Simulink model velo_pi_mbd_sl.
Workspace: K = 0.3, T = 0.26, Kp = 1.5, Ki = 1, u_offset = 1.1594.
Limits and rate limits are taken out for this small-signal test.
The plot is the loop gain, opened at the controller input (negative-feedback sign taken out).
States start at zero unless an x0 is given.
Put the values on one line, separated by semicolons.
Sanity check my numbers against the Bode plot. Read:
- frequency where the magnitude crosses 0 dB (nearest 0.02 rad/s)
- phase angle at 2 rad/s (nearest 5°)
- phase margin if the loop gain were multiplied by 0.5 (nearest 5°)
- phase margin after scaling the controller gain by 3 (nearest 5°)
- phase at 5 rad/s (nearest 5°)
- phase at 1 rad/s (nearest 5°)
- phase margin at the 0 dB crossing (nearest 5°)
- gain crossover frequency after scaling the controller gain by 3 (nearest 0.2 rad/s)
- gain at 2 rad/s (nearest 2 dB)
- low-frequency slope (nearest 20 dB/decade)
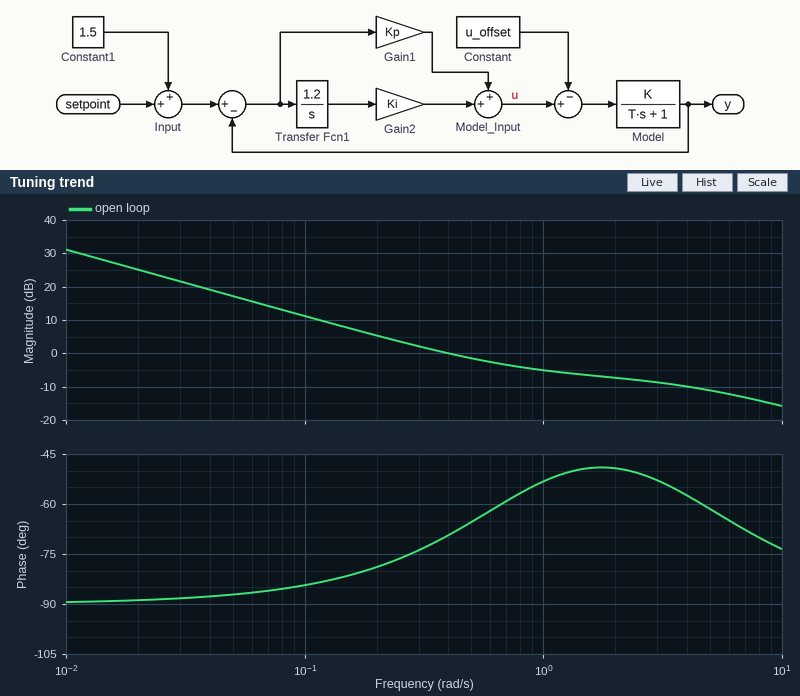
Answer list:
0.40 rad/s; -50°; 100°; 125°; -60°; -55°; 110°; 3.6 rad/s; -8 dB; -20 dB/decade
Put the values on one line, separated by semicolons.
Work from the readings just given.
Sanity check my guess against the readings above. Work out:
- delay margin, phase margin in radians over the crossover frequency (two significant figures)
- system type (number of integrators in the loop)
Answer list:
4.8 s; 1
